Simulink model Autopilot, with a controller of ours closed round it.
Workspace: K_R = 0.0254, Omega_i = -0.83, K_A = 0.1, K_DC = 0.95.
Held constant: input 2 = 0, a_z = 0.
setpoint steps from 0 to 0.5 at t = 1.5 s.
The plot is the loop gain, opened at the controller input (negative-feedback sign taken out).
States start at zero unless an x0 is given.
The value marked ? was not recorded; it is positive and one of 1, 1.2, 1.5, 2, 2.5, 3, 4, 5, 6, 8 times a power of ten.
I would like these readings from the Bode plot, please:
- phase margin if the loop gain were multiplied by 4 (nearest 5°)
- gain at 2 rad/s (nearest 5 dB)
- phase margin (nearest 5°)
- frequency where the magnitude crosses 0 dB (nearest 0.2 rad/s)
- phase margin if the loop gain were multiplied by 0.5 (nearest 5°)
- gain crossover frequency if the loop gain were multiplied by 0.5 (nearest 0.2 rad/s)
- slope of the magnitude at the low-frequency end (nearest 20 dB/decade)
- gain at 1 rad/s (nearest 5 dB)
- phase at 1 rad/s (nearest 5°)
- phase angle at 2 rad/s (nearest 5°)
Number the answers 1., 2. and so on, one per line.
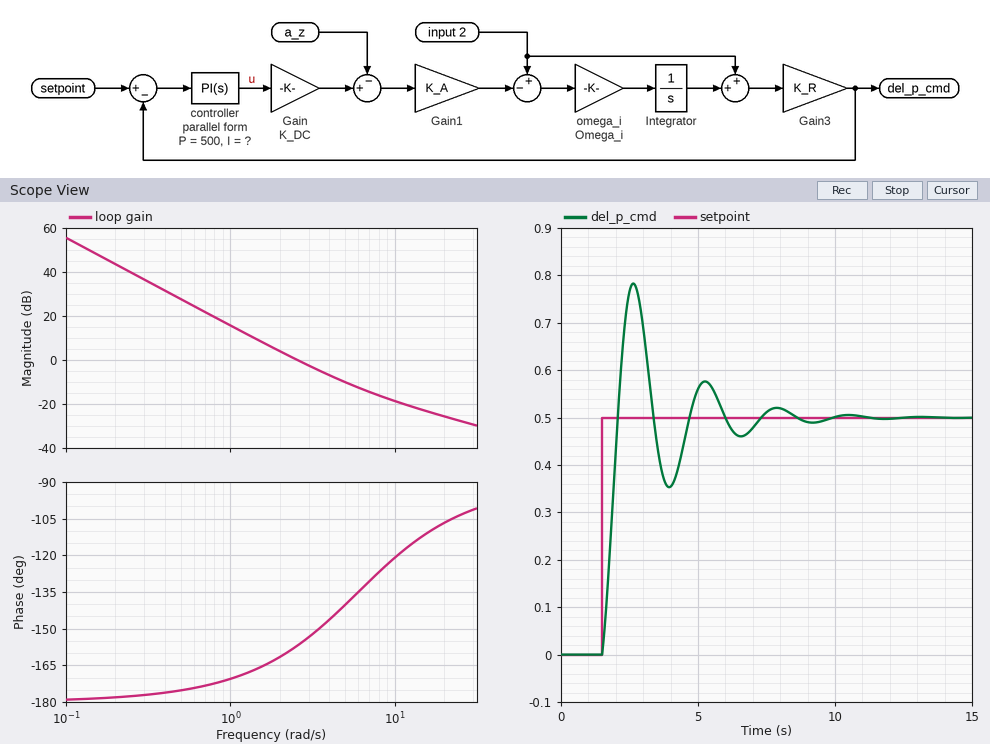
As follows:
1. 45°
2. 5 dB
3. 25°
4. 2.6 rad/s
5. 15°
6. 1.8 rad/s
7. -40 dB/decade
8. 15 dB
9. -170°
10. -160°
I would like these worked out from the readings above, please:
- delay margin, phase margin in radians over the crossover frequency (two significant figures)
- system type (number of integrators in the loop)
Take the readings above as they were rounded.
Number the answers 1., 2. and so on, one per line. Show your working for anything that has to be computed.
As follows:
1. 25 × π / 180 / 2.6 = 0.17 s
2. 2
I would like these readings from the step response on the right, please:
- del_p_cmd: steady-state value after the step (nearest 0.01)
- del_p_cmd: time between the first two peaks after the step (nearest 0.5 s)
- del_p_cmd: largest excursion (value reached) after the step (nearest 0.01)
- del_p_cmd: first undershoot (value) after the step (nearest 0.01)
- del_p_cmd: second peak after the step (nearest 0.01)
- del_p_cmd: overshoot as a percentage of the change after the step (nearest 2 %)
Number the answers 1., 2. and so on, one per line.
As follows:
1. 0.50
2. 2.5 s
3. 0.78
4. 0.35
5. 0.58
6. 56 %
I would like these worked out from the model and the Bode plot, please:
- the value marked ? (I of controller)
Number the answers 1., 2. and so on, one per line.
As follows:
1. 3000
